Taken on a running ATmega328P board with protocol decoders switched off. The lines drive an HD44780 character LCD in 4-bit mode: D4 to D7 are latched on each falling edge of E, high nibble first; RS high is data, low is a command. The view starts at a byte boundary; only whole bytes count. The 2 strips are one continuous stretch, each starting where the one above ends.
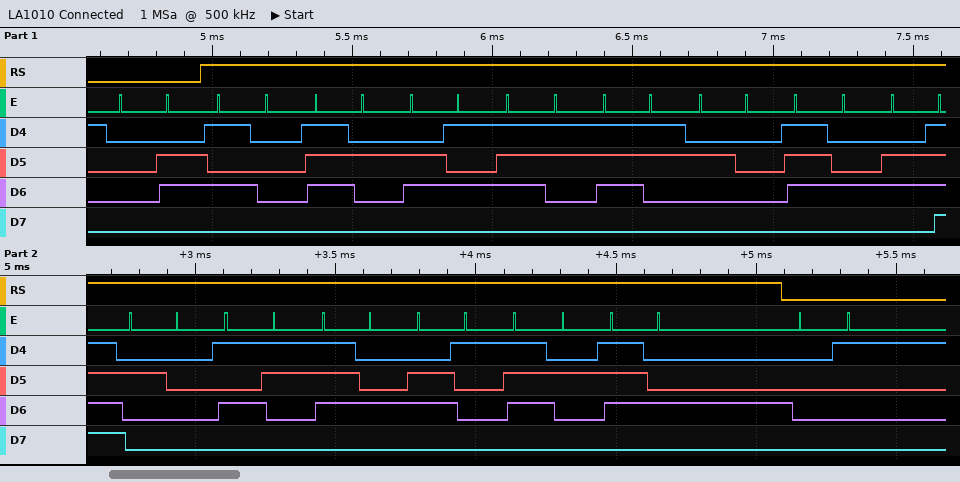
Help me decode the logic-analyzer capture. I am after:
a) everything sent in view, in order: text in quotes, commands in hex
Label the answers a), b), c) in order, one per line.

a) 0x06 "Press to Start" 0x01
